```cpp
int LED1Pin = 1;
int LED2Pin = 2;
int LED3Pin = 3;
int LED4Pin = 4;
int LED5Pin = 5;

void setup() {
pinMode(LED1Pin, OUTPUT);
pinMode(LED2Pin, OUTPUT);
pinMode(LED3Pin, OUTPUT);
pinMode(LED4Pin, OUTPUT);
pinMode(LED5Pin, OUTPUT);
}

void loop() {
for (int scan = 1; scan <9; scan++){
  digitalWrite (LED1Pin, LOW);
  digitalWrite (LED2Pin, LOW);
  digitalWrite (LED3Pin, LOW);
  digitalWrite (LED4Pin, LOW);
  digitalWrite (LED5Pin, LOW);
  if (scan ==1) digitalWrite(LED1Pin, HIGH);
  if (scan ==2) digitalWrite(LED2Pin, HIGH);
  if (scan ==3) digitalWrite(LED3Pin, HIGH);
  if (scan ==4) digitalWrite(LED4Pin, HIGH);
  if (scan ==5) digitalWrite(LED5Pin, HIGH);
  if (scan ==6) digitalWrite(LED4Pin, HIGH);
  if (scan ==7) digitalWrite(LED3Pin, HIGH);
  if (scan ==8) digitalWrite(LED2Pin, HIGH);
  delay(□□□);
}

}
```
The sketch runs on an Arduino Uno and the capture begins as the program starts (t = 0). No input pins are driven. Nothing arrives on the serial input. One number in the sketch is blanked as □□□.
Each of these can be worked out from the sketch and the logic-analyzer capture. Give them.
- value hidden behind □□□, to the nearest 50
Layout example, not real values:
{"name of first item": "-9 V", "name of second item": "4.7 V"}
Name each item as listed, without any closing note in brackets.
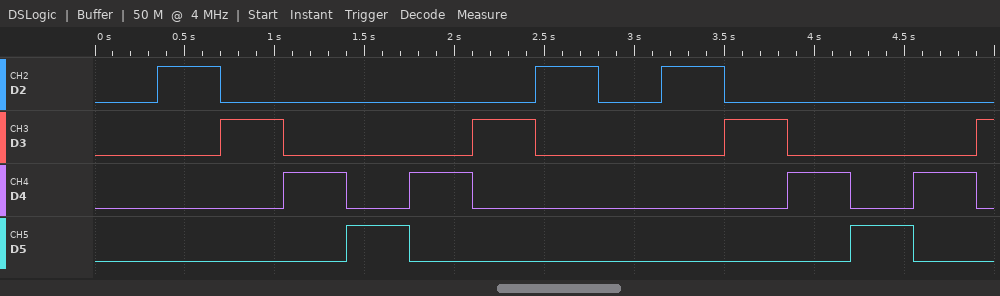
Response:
{"value hidden behind □□□, to the nearest 50": "350"}
